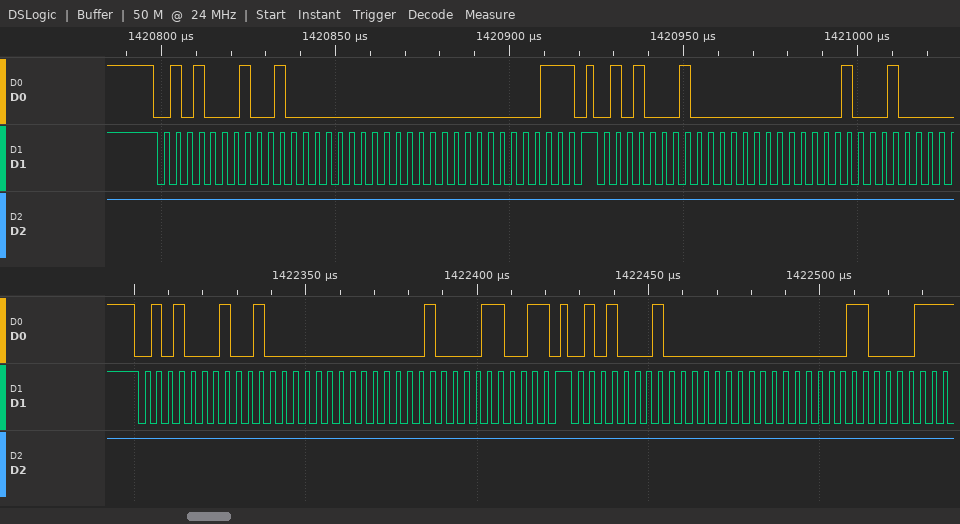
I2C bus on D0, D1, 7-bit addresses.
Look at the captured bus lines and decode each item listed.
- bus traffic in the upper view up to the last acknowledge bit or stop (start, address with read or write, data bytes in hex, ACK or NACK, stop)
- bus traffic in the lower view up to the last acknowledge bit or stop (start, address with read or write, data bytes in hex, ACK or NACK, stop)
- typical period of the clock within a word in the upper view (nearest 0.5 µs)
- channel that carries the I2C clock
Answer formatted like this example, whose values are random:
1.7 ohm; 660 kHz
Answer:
start, address 28 read ACK, 40 ACK, 00 ACK, 03 NACK, stop, start, address 28 read ACK, 00 ACK, 11 ACK; start, address 28 read ACK, 40 ACK, 01 ACK, 19 NACK, stop, start, address 28 read ACK, 00 ACK, 03 ACK; 3.5 µs; D1
